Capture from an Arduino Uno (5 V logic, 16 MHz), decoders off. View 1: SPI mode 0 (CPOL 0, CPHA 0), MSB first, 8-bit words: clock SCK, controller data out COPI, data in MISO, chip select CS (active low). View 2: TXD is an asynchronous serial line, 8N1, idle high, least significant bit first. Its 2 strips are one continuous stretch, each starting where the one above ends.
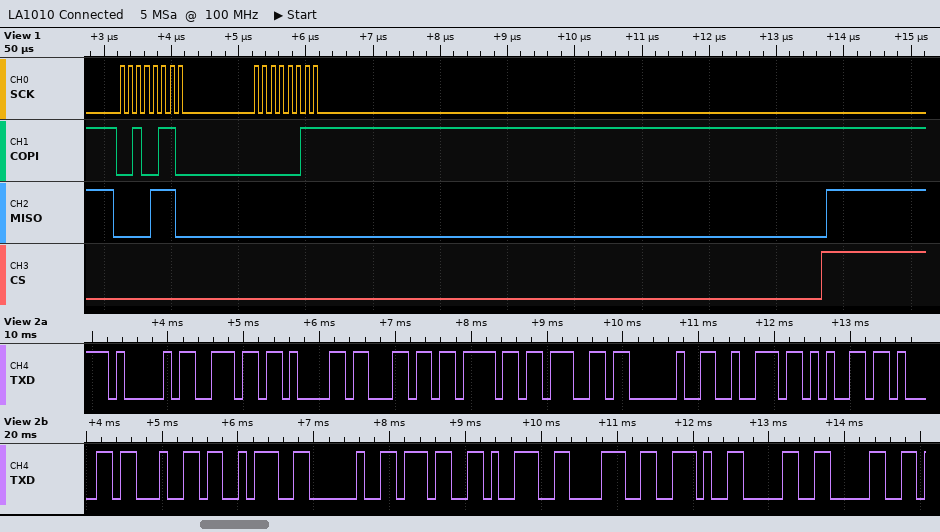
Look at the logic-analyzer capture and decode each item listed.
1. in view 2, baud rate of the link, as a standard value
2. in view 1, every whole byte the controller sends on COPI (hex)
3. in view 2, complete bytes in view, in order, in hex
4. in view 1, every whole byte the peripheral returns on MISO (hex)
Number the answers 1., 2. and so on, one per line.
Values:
1. 9600 baud
2. 26 03
3. 0x41 0x6E 0x61 0x6C 0x6F 0x67 0x20 0x72 0x65 0x61 0x64 0x3A 0x20 0x37 0x39 0x38 0x2E 0x30 0x30
4. 0E 00
